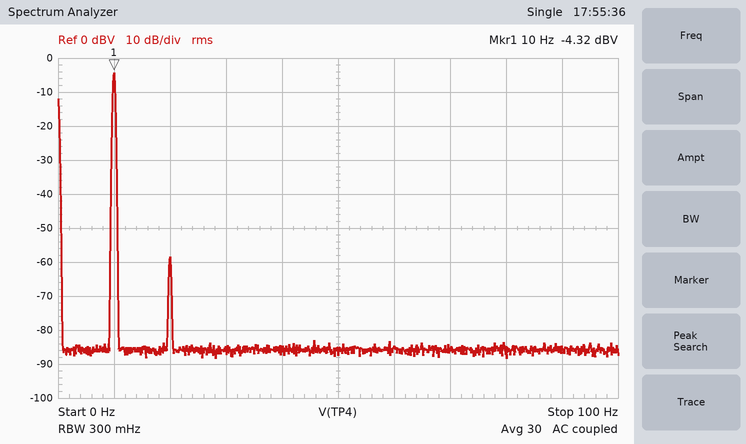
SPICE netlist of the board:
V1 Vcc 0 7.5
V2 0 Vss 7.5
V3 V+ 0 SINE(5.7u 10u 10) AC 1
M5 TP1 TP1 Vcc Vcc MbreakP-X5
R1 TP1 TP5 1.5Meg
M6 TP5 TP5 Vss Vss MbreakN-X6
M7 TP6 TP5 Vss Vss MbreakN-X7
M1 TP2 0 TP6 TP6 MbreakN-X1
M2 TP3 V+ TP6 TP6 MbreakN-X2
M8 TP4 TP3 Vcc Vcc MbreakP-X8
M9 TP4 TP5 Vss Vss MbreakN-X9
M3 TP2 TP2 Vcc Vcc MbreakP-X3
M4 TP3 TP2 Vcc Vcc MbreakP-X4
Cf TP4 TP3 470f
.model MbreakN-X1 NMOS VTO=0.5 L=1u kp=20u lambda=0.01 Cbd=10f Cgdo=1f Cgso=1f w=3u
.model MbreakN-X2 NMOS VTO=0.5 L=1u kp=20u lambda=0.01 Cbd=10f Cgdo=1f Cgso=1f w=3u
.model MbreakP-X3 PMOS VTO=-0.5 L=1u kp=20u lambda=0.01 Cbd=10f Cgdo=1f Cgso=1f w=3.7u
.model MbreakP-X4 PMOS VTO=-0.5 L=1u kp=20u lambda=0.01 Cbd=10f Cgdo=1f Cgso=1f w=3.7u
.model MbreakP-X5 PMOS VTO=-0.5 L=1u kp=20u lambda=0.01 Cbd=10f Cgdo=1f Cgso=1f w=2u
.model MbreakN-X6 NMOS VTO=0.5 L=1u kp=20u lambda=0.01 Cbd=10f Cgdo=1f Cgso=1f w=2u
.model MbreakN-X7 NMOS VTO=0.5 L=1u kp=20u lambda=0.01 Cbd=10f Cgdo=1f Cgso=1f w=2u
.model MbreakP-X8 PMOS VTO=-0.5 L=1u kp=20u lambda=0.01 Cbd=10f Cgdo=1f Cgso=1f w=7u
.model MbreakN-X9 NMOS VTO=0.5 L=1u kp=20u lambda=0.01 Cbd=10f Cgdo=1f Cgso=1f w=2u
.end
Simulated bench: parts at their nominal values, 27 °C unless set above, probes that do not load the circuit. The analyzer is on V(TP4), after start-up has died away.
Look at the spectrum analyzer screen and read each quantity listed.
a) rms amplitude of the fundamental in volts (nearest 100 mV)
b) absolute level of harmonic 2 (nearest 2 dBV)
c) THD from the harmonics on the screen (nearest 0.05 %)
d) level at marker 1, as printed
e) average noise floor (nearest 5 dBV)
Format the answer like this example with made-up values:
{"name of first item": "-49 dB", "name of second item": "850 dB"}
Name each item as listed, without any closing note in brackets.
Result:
{"rms amplitude of the fundamental in volts": "600 mV", "absolute level of harmonic 2": "-58 dBV", "THD from the harmonics on the screen": "0.20 %", "level at marker 1, as printed": "-4.32 dBV", "average noise floor": "-85 dBV"}
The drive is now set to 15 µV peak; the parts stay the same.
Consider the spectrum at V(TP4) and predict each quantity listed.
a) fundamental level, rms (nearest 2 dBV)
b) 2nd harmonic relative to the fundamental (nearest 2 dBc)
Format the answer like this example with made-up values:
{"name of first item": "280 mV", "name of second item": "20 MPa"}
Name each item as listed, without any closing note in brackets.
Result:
{"fundamental level, rms": "0 dBV", "2nd harmonic relative to the fundamental": "-50 dBc"}
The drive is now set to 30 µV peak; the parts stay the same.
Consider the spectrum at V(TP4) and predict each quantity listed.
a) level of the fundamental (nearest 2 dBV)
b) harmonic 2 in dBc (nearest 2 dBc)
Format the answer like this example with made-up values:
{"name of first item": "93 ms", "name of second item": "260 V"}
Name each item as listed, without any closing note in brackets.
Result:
{"level of the fundamental": "6 dBV", "harmonic 2 in dBc": "-44 dBc"}
